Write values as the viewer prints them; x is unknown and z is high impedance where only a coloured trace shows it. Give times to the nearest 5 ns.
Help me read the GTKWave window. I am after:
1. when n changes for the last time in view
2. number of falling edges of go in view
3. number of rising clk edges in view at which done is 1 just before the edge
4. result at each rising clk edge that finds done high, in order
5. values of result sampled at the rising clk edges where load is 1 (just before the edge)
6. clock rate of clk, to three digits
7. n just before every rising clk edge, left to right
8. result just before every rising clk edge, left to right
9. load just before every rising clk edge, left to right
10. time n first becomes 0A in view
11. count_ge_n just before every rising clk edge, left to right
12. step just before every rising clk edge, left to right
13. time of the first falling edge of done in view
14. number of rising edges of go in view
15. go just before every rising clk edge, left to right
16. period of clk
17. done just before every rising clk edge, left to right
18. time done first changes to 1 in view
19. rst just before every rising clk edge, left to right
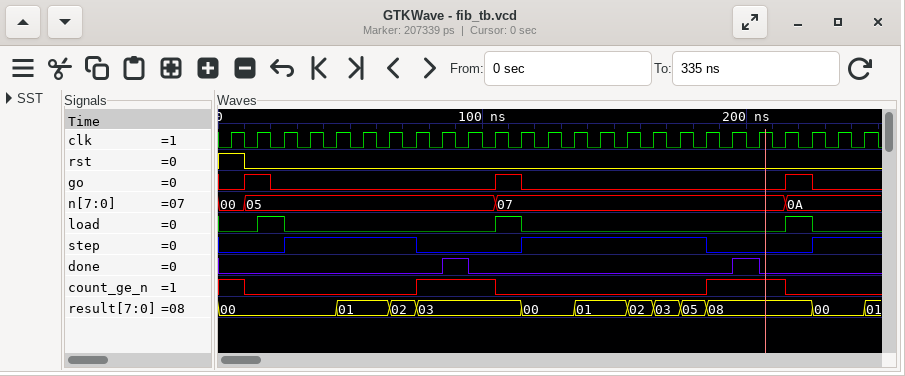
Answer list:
215 ns
3
2
03, 08
00, 03, 08
100 MHz
00, 05, 05, 05, 05, 05, 05, 05, 05, 05, 05, 07, 07, 07, 07, 07, 07, 07, 07, 07, 07, 07, 0A, 0A, 0A
00, 00, 00, 00, 00, 01, 01, 02, 03, 03, 03, 03, 00, 00, 01, 01, 02, 03, 05, 08, 08, 08, 08, 00, 00
0 0 1 0 0 0 0 0 0 0 0 1 0 0 0 0 0 0 0 0 0 0 1 0 0
215 ns
1 0 0 0 0 0 0 0 1 1 1 0 0 0 0 0 0 0 0 1 1 1 0 0 0
0 0 0 1 1 1 1 1 0 0 0 0 1 1 1 1 1 1 1 0 0 0 0 1 1
95 ns
3
0 1 0 0 0 0 0 0 0 0 0 1 0 0 0 0 0 0 0 0 0 0 1 0 0
10 ns
0 0 0 0 0 0 0 0 0 1 0 0 0 0 0 0 0 0 0 0 1 0 0 0 0
85 ns
1 0 0 0 0 0 0 0 0 0 0 0 0 0 0 0 0 0 0 0 0 0 0 0 0
